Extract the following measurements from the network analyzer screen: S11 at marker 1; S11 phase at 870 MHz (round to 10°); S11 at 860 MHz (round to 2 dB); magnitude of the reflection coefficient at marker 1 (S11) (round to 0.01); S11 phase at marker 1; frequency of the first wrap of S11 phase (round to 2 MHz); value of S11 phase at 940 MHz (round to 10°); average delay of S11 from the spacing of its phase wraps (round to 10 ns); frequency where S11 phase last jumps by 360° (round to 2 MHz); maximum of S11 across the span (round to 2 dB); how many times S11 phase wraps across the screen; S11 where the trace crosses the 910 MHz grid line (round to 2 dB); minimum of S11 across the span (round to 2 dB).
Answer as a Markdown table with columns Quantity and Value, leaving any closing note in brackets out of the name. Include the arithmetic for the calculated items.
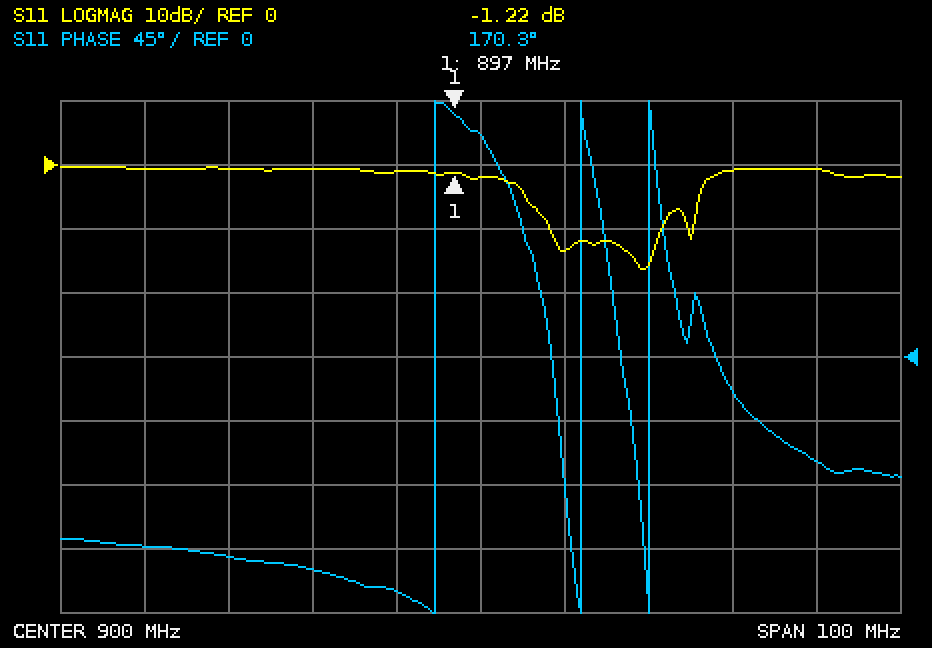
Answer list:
| Quantity | Value |
|---|---|
| S11 at marker 1 | -1.22 dB |
| S11 phase at 870 MHz | -140° |
| S11 at 860 MHz | 0 dB |
| magnitude of the reflection coefficient at marker 1 (S11) | 10^(-1.22/20) ≈ 0.87 |
| S11 phase at marker 1 | 170.3° |
| frequency of the first wrap of S11 phase | 894 MHz |
| value of S11 phase at 940 MHz | -70° |
| average delay of S11 from the spacing of its phase wraps | 2 cycles / (920 MHz − 894 MHz) ≈ 76.9 ns, so 80 ns to the nearest 10 ns |
| frequency where S11 phase last jumps by 360° | 920 MHz |
| maximum of S11 across the span | 0 dB |
| how many times S11 phase wraps across the screen | 3 |
| S11 where the trace crosses the 910 MHz grid line | -14 dB |
| minimum of S11 across the span | -16 dB |
